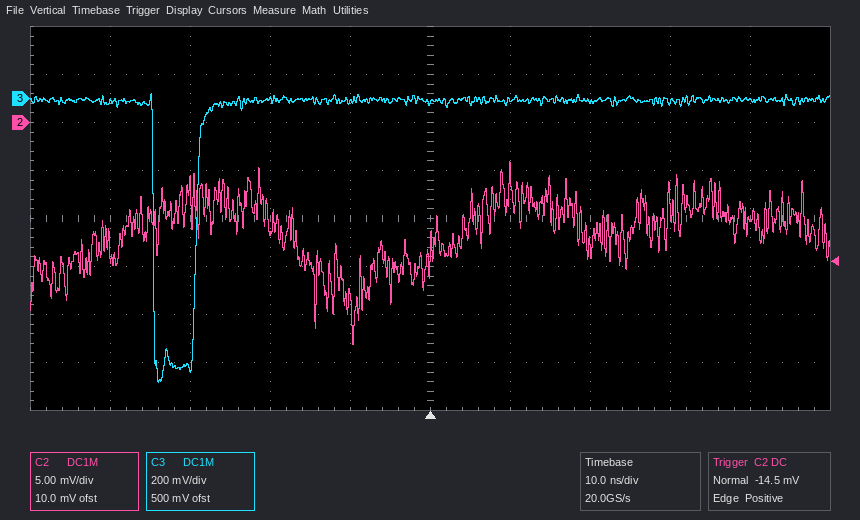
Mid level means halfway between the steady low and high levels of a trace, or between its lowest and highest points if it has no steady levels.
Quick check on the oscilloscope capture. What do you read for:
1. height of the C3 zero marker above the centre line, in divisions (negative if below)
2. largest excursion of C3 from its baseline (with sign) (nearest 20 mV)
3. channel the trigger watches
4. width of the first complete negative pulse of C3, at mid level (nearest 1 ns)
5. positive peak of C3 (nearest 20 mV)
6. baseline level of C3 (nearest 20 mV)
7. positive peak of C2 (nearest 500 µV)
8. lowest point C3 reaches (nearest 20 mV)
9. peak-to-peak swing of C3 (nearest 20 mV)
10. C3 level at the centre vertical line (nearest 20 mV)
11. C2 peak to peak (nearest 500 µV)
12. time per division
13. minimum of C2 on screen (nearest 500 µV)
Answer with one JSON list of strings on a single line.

["+2.5 div", "-1.18 V", "C2", "5 ns", "20 mV", "0 mV", "-4.0 mV", "-1.18 V", "1.20 V", "-20 mV", "19.0 mV", "10 ns", "-23.0 mV"]
